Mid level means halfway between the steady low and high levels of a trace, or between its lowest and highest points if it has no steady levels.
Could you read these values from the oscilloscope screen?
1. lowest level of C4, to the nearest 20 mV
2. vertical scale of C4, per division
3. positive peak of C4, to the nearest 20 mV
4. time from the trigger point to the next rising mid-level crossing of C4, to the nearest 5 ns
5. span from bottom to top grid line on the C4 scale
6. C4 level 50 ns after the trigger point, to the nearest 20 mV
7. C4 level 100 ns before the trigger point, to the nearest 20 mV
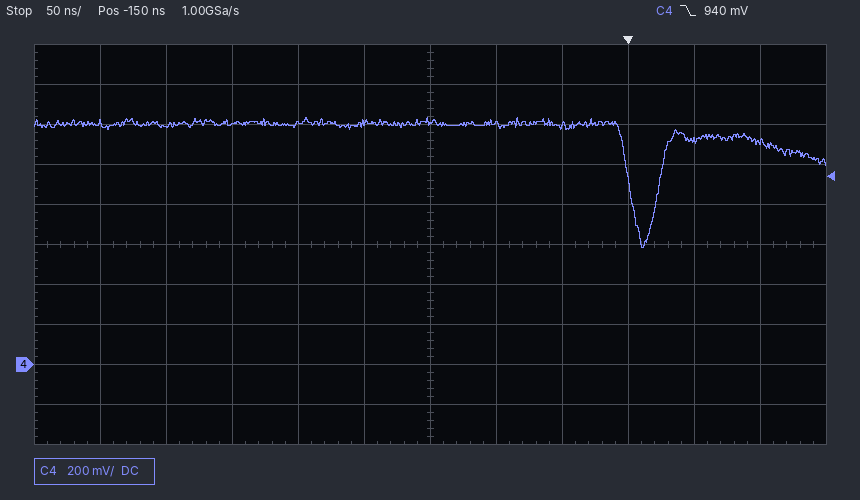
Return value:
580 mV
200 mV
1.24 V
25 ns
2 V
1.12 V
1.20 V
